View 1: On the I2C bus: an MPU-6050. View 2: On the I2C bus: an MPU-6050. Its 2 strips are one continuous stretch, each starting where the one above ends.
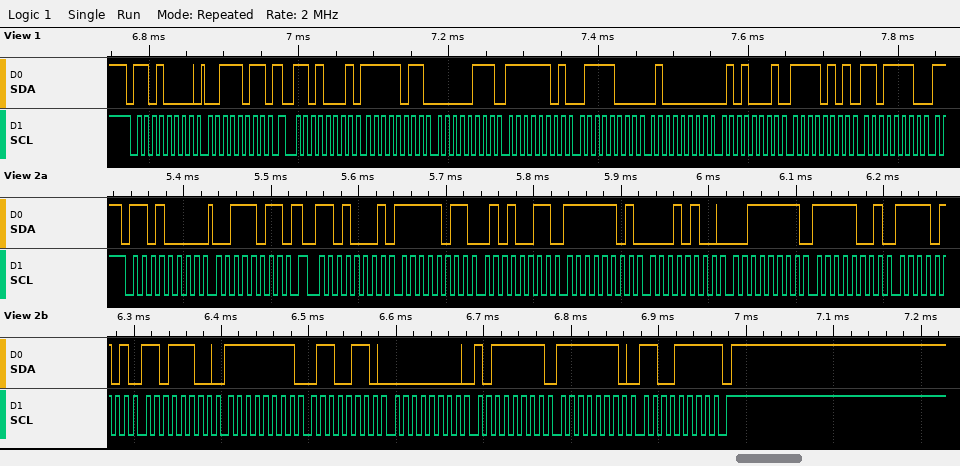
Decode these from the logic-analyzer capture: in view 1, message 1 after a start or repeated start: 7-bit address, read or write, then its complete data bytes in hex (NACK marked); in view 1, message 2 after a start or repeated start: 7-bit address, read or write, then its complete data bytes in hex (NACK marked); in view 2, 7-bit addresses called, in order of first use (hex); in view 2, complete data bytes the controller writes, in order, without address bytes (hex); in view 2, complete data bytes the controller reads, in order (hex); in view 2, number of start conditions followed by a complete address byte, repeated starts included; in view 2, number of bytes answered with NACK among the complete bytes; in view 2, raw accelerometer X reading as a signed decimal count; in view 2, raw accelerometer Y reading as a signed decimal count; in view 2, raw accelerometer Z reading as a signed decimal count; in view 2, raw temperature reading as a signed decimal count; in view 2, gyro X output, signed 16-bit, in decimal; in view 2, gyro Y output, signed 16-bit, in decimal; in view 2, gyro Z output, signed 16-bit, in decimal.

0x68 write: 3B
0x68 read: FB 07 FD 78 40 51 F5 DE
0x68
3B
FB 53 FD 14 3F F9 F5 DC FF 66 00 BF FE CF
2
1
-1197
-748
16377
-2596
-154
191
-305
